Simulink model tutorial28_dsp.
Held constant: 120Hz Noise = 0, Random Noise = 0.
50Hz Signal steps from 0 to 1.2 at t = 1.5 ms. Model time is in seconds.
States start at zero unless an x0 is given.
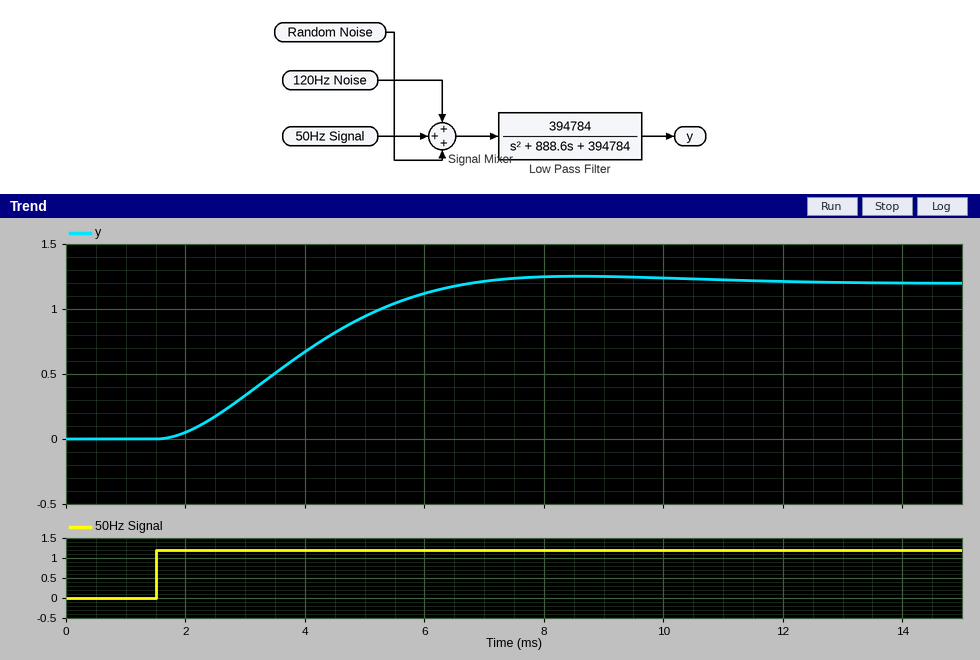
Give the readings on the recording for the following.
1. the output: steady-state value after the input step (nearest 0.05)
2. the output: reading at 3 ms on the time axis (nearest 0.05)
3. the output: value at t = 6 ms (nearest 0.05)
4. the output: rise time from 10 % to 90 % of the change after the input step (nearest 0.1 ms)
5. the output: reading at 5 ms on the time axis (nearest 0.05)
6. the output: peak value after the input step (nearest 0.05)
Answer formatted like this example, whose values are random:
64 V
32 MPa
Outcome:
1.20
0.35
1.10
3.4 ms
0.95
1.25
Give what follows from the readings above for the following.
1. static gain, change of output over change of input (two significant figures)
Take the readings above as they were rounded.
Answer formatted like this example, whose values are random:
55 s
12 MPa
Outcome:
1.0
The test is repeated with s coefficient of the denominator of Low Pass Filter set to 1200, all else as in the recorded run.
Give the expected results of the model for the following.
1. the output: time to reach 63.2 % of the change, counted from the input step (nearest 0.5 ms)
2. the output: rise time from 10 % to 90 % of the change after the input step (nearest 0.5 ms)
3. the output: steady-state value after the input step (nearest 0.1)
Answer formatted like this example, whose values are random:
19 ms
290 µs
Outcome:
3.5 ms
5.0 ms
1.2
